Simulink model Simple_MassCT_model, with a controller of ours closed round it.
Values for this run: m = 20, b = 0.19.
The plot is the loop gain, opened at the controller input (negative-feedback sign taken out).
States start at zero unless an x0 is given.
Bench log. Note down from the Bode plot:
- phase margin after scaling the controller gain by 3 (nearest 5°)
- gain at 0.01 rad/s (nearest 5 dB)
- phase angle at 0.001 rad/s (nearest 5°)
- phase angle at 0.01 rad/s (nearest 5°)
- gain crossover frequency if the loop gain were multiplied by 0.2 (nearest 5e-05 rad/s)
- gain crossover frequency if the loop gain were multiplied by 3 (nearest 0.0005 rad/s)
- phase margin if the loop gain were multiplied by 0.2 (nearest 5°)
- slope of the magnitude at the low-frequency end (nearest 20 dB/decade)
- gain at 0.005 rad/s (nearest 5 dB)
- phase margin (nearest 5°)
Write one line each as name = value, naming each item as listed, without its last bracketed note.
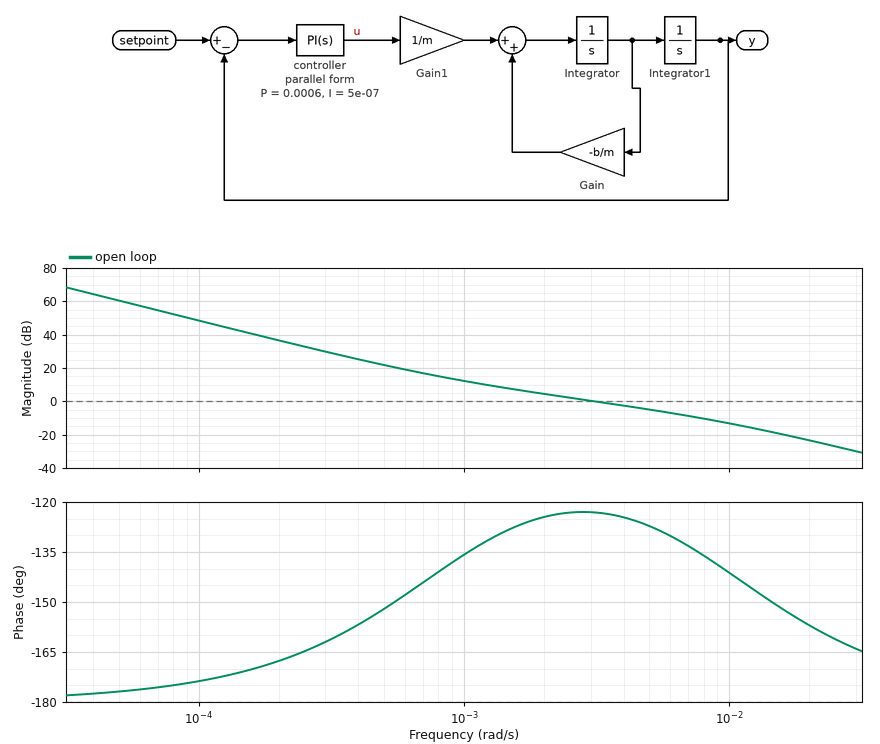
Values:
phase margin after scaling the controller gain by 3 = 45°
gain at 0.01 rad/s = -15 dB
phase angle at 0.001 rad/s = -135°
phase angle at 0.01 rad/s = -140°
gain crossover frequency if the loop gain were multiplied by 0.2 = 0.00085 rad/s
gain crossover frequency if the loop gain were multiplied by 3 = 0.0075 rad/s
phase margin if the loop gain were multiplied by 0.2 = 40°
slope of the magnitude at the low-frequency end = -40 dB/decade
gain at 0.005 rad/s = -5 dB
phase margin = 55°
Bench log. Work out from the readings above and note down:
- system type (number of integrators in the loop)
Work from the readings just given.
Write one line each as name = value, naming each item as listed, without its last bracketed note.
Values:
system type = 2
